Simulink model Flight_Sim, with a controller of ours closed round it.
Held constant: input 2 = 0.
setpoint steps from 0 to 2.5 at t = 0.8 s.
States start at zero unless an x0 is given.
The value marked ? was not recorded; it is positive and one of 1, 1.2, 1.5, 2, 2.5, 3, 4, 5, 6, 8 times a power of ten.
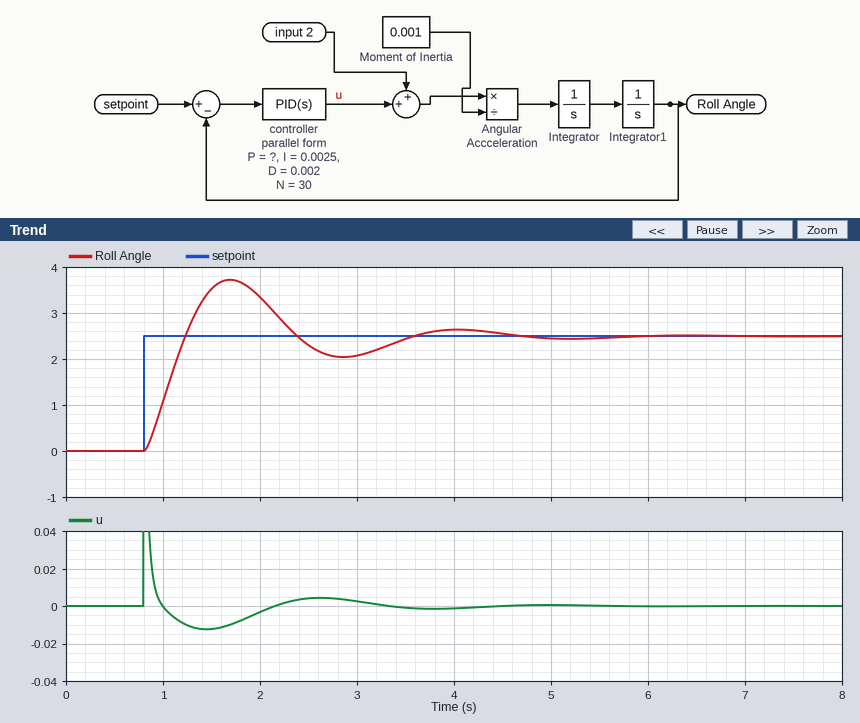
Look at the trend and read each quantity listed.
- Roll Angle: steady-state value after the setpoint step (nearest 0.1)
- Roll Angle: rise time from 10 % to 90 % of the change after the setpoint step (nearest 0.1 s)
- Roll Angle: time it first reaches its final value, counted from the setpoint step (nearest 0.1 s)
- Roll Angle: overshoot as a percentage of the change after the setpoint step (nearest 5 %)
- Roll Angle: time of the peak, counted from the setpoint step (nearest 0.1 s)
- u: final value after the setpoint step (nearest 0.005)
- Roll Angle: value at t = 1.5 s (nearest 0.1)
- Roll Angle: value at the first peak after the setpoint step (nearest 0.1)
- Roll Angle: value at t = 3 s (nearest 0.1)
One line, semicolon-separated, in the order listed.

2.5; 0.3 s; 0.4 s; 50 %; 0.9 s; 0.000; 3.5; 3.7; 2.1
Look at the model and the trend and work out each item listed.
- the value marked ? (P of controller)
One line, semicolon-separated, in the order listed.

0.008
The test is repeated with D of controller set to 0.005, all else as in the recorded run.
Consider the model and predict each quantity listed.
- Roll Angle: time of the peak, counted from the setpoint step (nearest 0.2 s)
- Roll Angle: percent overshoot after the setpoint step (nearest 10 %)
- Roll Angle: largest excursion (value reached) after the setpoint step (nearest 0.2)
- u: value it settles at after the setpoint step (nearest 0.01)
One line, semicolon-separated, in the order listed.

0.6 s; 20 %; 3.0; 0.00
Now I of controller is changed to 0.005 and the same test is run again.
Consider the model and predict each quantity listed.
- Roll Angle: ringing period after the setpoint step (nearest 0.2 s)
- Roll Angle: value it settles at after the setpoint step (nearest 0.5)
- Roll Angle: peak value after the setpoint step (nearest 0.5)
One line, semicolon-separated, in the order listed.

2.4 s; 2.5; 4.0
